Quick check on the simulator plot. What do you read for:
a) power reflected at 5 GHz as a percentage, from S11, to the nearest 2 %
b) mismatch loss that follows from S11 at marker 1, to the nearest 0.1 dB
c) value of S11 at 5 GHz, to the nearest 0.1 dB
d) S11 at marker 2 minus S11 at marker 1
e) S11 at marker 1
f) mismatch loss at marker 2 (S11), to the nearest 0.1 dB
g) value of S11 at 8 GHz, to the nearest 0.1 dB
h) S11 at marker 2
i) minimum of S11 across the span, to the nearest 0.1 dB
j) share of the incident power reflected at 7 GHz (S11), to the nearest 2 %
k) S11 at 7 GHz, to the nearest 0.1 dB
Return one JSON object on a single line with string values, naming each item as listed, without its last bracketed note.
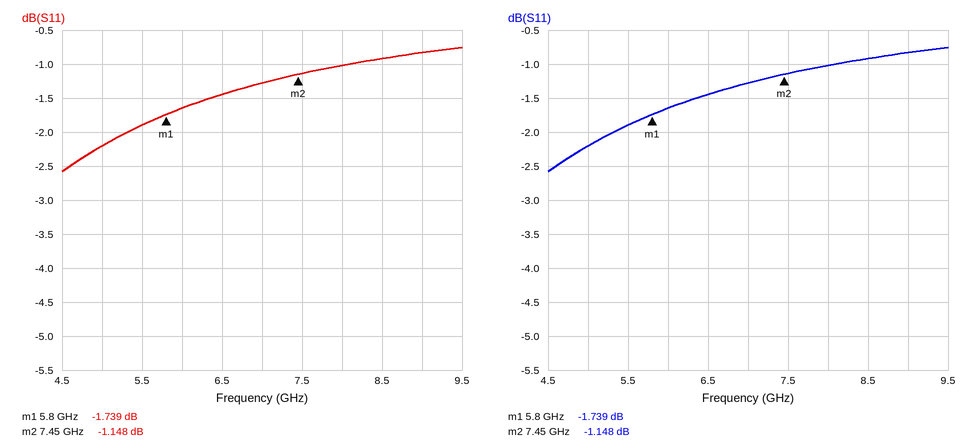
{"power reflected at 5 GHz as a percentage, from S11, to the nearest 2 %": "60 %", "mismatch loss that follows from S11 at marker 1, to the nearest 0.1 dB": "4.8 dB", "value of S11 at 5 GHz, to the nearest 0.1 dB": "-2.2 dB", "S11 at marker 2 minus S11 at marker 1": "0.591 dB", "S11 at marker 1": "-1.739 dB", "mismatch loss at marker 2 (S11), to the nearest 0.1 dB": "6.3 dB", "value of S11 at 8 GHz, to the nearest 0.1 dB": "-1.0 dB", "S11 at marker 2": "-1.148 dB", "minimum of S11 across the span, to the nearest 0.1 dB": "-2.6 dB", "share of the incident power reflected at 7 GHz (S11), to the nearest 2 %": "74 %", "S11 at 7 GHz, to the nearest 0.1 dB": "-1.3 dB"}
